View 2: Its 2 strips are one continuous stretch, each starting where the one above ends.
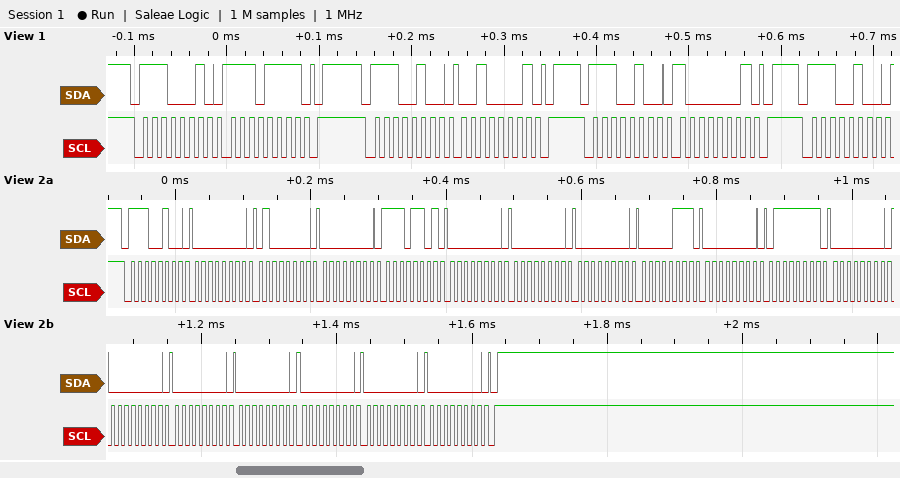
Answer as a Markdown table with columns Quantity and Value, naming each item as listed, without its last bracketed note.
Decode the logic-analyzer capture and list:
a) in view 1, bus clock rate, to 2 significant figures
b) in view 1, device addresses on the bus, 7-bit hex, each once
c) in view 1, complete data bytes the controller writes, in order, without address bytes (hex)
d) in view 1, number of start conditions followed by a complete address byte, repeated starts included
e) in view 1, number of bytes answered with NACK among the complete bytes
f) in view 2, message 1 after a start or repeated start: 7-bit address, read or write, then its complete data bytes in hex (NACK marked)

| Quantity | Value |
|---|---|
| in view 1, bus clock rate, to 2 significant figures | 100 kHz |
| in view 1, device addresses on the bus, 7-bit hex, each once | 0x71 0x72 |
| in view 1, complete data bytes the controller writes, in order, without address bytes | EF 21 81 |
| in view 1, number of start conditions followed by a complete address byte, repeated starts included | 4 |
| in view 1, number of bytes answered with NACK among the complete bytes | 0 |
| in view 2, message 1 after a start or repeated start: 7-bit address, read or write, then its complete data bytes in hex | 0x72 write: 00 40 00 ED 00 00 00 07 00 7F 00 00 00 00 00 00 00 |
